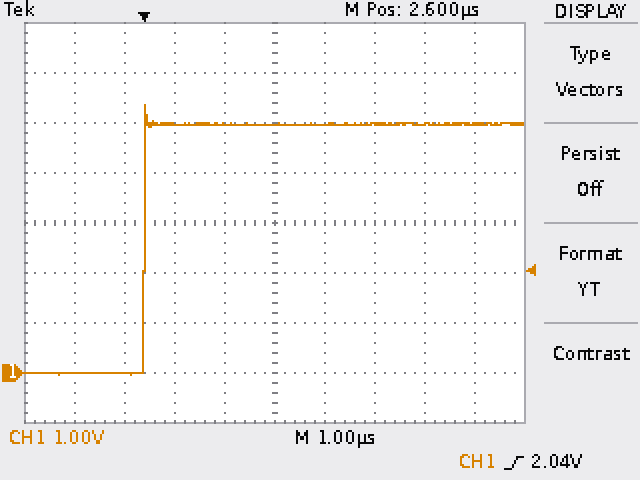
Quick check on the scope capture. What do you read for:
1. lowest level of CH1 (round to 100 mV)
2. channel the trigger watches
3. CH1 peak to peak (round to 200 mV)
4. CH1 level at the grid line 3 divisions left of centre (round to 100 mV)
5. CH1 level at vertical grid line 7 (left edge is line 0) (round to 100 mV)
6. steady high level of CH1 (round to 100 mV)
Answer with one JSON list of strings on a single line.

["0.0 V", "CH1", "5.4 V", "0.0 V", "5.0 V", "5.0 V"]
